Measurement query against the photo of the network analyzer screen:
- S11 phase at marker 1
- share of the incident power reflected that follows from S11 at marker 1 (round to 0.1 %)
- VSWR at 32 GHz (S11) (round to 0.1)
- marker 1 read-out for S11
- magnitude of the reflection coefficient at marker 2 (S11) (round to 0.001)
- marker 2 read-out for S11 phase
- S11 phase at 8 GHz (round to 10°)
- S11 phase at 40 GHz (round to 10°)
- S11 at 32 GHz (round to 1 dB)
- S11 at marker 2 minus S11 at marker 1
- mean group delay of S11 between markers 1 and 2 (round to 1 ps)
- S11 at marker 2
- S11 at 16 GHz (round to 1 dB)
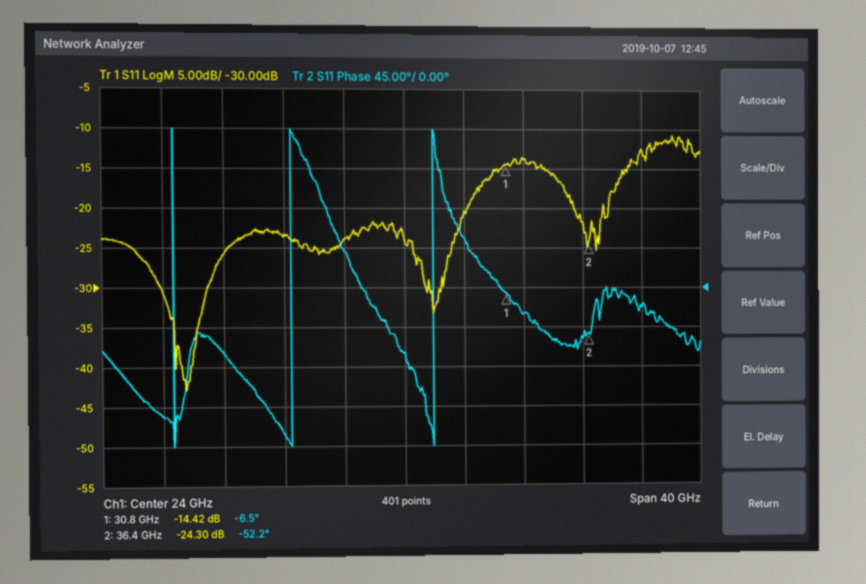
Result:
-6.5°
3.6 %
1.5
-14.42 dB
0.061
-52.2°
-150°
-20°
-14 dB
-9.88 dB
23 ps
-24.30 dB
-23 dB
